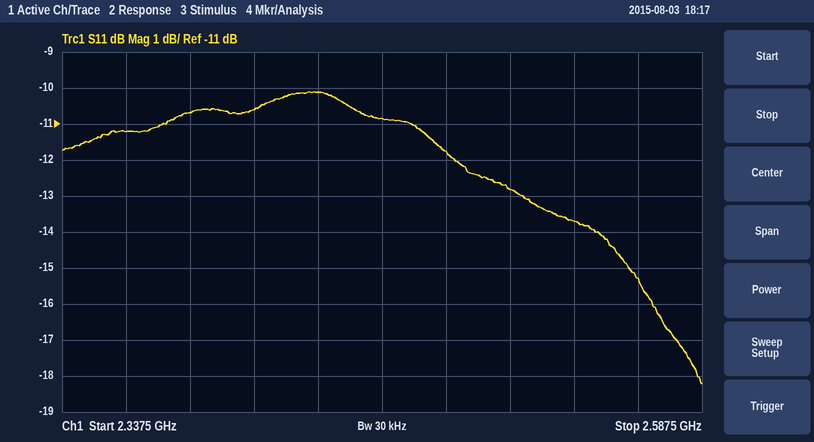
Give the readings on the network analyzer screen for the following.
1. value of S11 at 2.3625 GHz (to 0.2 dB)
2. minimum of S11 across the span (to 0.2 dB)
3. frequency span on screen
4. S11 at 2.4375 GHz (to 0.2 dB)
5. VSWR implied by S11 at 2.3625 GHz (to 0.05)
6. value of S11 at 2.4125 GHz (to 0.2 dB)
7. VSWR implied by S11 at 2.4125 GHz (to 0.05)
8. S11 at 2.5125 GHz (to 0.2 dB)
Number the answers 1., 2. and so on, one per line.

1. -11.2 dB
2. -18.2 dB
3. 250 MHz
4. -10.2 dB
5. 1.75
6. -10.6 dB
7. 1.85
8. -12.8 dB
